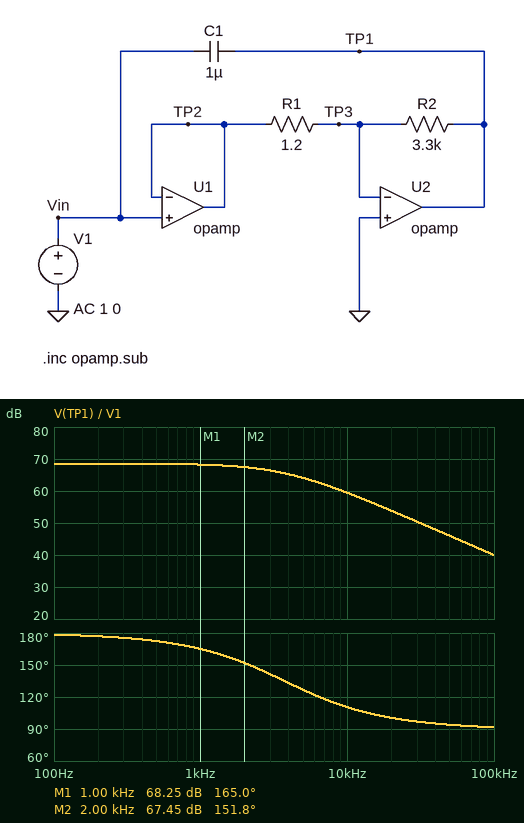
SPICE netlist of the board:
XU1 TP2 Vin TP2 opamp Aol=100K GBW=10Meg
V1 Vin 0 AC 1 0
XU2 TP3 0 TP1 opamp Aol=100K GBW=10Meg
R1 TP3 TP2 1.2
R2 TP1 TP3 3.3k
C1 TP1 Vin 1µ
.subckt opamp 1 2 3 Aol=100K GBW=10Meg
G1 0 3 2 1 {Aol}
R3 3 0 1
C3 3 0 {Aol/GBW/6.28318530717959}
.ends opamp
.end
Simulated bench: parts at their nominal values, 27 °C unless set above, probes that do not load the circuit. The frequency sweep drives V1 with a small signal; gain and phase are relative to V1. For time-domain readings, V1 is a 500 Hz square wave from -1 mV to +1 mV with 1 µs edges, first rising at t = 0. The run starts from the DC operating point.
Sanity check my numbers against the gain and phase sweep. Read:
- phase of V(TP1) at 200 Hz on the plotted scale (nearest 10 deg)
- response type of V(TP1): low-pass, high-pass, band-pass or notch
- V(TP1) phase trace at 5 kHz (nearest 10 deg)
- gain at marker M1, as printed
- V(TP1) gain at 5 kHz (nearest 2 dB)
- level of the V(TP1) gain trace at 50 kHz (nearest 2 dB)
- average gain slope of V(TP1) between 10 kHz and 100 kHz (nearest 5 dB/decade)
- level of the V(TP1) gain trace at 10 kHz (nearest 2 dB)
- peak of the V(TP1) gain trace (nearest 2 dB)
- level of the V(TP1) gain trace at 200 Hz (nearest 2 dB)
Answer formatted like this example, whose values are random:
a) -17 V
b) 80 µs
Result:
a) 180 deg
b) low-pass
c) 130 deg
d) 68.25 dB
e) 64 dB
f) 46 dB
g) -20 dB/decade
h) 60 dB
i) 68 dB
j) 68 dB
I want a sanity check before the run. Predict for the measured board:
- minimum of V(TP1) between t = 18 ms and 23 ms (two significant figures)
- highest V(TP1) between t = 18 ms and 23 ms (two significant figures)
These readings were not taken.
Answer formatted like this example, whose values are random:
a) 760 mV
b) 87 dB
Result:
a) -2.7 V
b) 2.7 V
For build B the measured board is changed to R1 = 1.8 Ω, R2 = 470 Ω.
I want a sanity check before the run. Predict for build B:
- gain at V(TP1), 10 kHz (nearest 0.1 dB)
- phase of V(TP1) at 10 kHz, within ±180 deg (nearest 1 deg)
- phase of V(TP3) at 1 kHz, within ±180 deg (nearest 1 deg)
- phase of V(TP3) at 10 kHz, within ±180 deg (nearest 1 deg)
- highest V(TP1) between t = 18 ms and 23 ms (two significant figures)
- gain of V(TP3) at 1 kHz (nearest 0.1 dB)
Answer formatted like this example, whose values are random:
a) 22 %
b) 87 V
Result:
a) 48.0 dB
b) 165 deg
c) 83 deg
d) 75 deg
e) 260 mV
f) -31.6 dB
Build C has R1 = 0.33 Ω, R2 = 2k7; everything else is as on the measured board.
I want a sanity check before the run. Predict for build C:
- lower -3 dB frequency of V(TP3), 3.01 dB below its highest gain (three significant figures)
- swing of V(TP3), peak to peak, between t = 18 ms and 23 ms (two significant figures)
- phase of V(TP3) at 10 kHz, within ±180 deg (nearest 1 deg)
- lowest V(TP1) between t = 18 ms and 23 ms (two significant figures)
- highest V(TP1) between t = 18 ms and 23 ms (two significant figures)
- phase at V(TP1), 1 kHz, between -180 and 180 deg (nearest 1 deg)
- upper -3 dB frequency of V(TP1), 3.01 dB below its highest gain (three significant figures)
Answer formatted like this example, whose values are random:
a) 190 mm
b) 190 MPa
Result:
a) 1.31 kHz
b) 3.8 mV
c) 7 deg
d) -7.6 V
e) 7.6 V
f) 143 deg
g) 1.32 kHz
